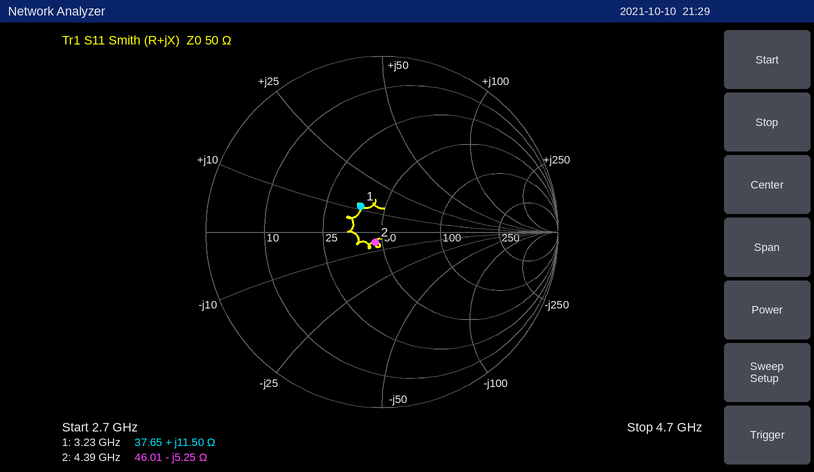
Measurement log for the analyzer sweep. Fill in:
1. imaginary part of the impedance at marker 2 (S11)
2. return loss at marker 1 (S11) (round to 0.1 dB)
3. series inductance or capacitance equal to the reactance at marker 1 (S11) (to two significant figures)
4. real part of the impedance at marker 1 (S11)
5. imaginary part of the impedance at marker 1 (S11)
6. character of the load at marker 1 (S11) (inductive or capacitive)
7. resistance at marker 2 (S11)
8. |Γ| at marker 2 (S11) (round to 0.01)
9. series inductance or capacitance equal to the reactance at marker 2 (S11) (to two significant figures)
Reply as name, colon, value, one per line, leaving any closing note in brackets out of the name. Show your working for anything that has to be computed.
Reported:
imaginary part of the impedance at marker 2: -5.25 Ω
return loss at marker 1 (S11): 14.4 dB
series inductance or capacitance equal to the reactance at marker 1 (S11): L = 11.5 Ω/(2π × 3.23 GHz) ≈ 567 pH, so 570 pH to two significant figures
real part of the impedance at marker 1: 37.65 Ω
imaginary part of the impedance at marker 1: +11.50 Ω
character of the load at marker 1 (S11): inductive
resistance at marker 2: 46.01 Ω
|Γ| at marker 2 (S11): 0.07
series inductance or capacitance equal to the reactance at marker 2 (S11): C = 1/(2π × 4.39 GHz × 5.25 Ω) ≈ 6.9 pF
